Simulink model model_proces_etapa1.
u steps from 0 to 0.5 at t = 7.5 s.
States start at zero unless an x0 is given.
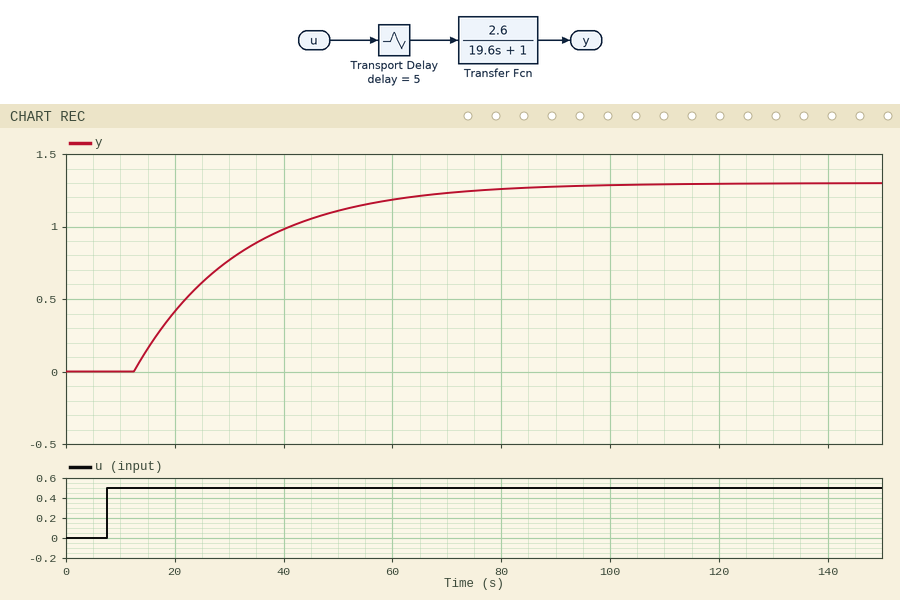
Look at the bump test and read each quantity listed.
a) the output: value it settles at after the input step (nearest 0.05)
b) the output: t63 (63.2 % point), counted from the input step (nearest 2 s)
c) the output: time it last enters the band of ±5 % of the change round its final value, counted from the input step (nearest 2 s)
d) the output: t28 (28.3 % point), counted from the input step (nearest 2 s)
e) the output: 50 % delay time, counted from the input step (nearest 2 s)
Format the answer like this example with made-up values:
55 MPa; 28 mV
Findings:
1.30; 24 s; 64 s; 12 s; 18 s
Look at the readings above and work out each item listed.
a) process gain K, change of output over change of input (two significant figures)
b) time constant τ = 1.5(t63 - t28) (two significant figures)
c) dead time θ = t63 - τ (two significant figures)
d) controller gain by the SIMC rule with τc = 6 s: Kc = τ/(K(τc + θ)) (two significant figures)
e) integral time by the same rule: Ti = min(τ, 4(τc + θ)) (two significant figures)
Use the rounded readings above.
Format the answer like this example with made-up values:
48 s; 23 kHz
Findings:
2.6; 18 s; 6.0 s; 0.58; 18 s
